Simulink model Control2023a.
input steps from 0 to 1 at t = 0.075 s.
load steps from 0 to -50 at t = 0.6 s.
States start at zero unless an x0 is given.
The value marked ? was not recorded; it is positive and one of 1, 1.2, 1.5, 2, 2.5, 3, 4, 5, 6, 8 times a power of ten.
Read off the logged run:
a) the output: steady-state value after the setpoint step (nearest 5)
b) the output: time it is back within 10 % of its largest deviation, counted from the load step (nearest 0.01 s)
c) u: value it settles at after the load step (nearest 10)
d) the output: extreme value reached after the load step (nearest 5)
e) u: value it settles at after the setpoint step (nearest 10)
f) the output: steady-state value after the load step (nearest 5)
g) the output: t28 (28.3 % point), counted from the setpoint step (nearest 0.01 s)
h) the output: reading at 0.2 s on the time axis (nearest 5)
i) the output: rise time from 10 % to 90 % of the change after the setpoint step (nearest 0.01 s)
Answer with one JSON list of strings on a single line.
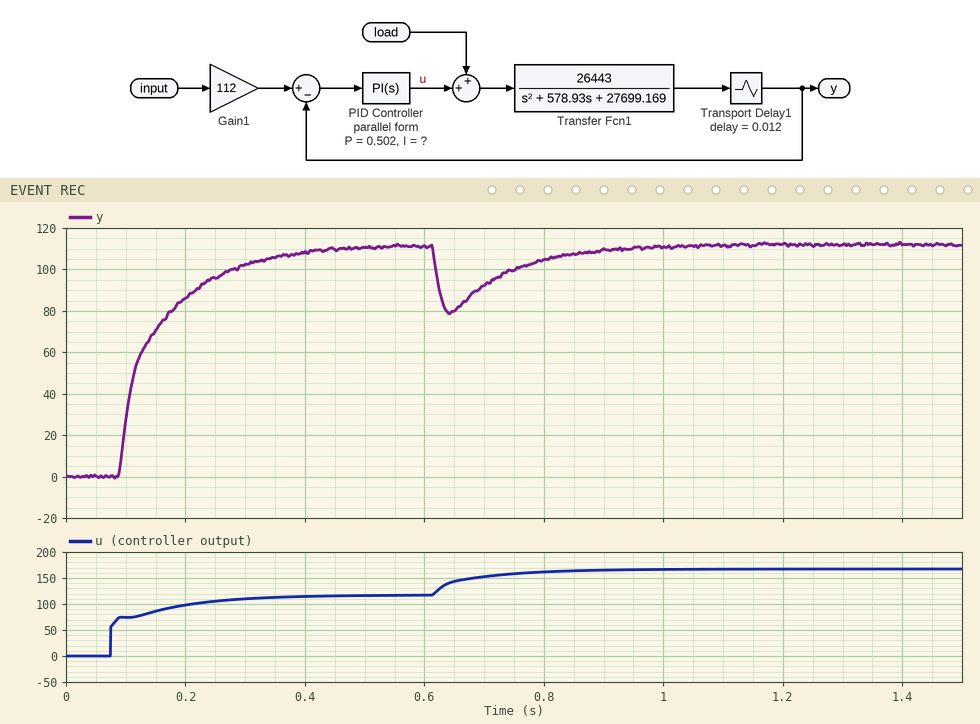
["110", "0.29 s", "170", "80", "120", "110", "0.03 s", "85", "0.19 s"]
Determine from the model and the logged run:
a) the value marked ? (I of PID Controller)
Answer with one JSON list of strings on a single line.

["12"]
